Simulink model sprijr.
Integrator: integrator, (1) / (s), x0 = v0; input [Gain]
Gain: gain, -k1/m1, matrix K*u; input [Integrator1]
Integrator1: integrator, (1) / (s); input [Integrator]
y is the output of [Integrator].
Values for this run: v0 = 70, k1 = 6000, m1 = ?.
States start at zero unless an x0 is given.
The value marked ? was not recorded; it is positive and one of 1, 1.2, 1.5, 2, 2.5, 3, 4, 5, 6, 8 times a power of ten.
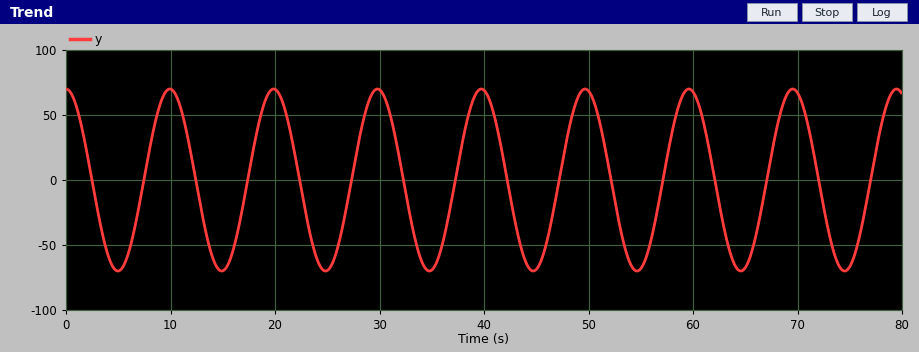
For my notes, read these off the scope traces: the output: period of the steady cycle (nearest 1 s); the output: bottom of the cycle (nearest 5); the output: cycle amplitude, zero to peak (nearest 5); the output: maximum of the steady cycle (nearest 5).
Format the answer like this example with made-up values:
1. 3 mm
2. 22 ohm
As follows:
1. 10 s
2. -70
3. 70
4. 70
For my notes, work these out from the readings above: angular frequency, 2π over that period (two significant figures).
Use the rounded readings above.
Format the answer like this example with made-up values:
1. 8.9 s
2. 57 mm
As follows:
1. 0.63 rad/s
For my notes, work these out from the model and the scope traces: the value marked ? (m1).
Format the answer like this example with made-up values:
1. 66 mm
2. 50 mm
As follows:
1. 15000
